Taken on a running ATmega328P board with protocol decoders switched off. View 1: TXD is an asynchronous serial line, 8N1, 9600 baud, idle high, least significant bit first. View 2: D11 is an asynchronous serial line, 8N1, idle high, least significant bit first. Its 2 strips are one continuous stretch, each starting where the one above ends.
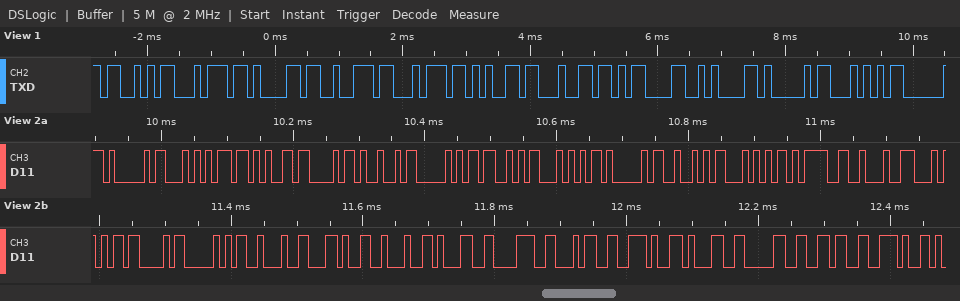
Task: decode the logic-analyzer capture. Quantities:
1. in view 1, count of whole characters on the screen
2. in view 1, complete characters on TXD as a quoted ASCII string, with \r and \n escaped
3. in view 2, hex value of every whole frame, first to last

11
"Started\r\nAT"
41 54 2B 43 49 50 53 54 41 52 54 3D 22 54 43 50 22 2C 22 31 38 34 2E 31 30 36 2E
